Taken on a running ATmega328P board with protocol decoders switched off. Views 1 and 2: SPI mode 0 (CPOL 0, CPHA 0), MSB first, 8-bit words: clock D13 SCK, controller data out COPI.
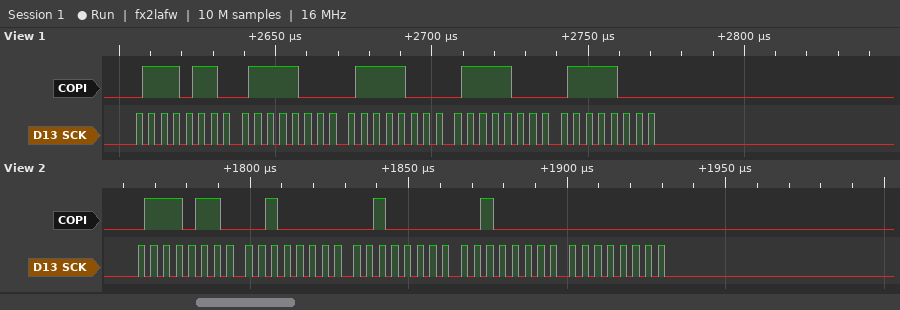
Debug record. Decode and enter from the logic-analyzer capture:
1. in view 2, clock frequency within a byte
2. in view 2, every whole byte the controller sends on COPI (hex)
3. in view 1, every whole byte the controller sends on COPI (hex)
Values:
250 kHz
0x76 0x20 0x20 0x20 0x00
0x76 0x78 0x78 0x78 0x78
